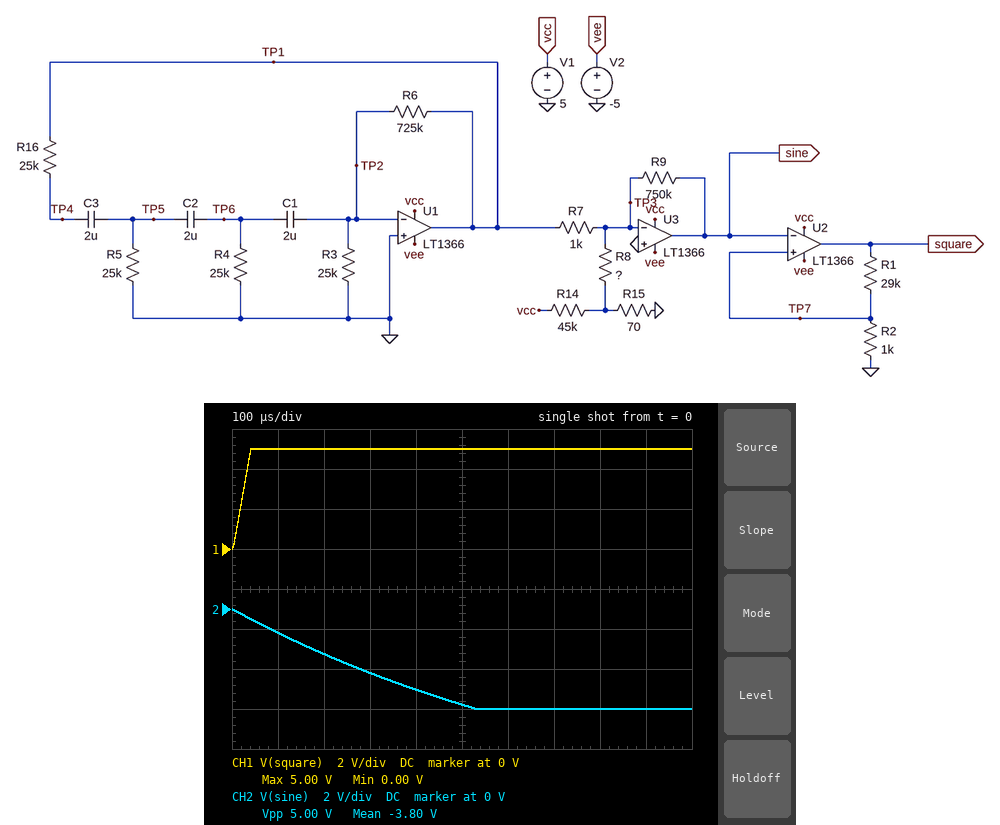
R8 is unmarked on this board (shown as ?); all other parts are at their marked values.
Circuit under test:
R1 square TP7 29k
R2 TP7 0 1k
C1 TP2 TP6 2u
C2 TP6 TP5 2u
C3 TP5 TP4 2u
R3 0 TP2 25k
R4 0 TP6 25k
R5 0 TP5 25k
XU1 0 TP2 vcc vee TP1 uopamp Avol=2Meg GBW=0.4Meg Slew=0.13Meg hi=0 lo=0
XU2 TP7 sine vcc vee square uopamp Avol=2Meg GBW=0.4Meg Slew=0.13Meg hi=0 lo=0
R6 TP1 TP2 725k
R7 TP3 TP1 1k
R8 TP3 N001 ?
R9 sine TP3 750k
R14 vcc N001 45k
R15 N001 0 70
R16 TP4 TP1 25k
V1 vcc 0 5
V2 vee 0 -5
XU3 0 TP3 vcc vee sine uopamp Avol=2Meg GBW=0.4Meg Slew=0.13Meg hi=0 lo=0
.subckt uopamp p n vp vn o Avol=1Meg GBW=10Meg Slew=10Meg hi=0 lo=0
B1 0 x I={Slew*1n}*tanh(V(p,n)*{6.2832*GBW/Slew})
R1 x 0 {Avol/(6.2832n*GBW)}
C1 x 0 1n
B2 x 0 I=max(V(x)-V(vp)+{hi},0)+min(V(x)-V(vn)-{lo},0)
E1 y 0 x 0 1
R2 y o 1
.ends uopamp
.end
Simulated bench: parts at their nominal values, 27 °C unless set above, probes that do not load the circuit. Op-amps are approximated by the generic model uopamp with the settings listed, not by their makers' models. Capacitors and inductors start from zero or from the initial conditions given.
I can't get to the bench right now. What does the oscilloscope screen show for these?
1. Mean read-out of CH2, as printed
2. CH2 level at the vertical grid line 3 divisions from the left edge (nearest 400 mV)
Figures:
-3.80 V
-3.2 V
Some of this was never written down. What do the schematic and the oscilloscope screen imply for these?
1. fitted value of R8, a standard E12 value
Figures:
470 Ω
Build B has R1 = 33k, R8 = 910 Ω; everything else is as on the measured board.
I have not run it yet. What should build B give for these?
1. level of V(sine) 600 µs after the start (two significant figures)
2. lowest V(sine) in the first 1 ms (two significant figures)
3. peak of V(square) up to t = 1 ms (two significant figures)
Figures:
-3.7 V
-4.8 V
5.0 V
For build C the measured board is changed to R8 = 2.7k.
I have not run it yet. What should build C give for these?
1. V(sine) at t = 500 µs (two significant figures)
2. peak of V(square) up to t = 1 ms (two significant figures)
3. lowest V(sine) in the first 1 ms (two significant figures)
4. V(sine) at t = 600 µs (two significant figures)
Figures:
-1.5 V
5.0 V
-1.9 V
-1.6 V
